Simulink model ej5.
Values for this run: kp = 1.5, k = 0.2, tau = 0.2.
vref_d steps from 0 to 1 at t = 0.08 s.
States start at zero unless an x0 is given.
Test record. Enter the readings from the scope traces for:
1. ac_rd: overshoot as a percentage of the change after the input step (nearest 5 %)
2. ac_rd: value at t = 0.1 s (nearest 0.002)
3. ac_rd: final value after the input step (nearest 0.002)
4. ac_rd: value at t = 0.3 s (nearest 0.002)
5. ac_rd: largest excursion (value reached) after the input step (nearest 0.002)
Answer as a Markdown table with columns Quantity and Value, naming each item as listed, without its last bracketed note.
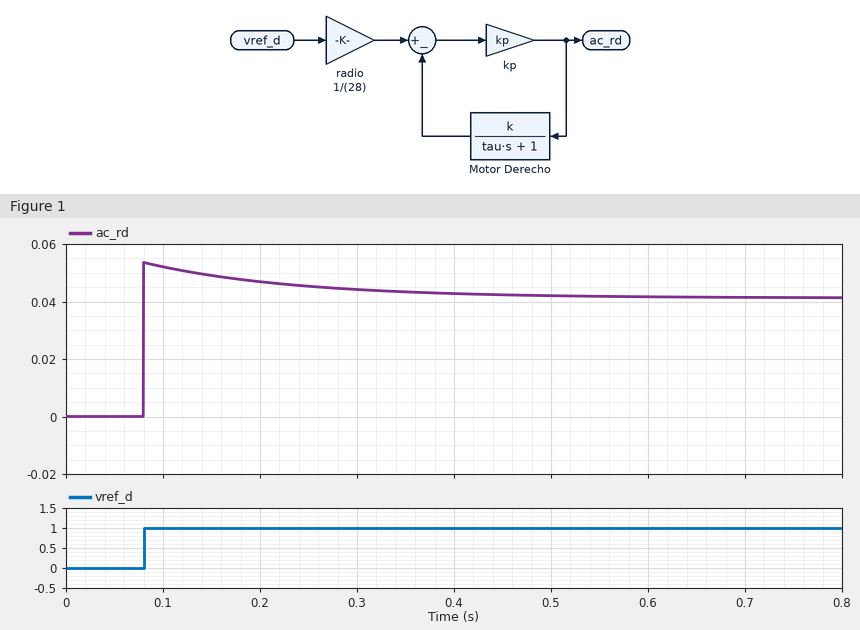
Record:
| Quantity | Value |
|---|---|
| ac_rd: overshoot as a percentage of the change after the input step | 30 % |
| ac_rd: value at t = 0.1 s | 0.052 |
| ac_rd: final value after the input step | 0.042 |
| ac_rd: value at t = 0.3 s | 0.044 |
| ac_rd: largest excursion (value reached) after the input step | 0.054 |
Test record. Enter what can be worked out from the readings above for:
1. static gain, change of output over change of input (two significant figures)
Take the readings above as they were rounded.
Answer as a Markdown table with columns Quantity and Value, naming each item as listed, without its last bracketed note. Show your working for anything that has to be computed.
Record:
| Quantity | Value |
|---|---|
| static gain, change of output over change of input | (0.042 - 0) / (1 - 0) = 0.042 |
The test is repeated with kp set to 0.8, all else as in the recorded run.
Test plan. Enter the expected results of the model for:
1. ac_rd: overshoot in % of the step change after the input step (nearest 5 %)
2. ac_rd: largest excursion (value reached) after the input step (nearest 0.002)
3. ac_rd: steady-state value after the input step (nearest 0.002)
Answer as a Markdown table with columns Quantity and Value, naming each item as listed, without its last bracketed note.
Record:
| Quantity | Value |
|---|---|
| ac_rd: overshoot in % of the step change after the input step | 15 % |
| ac_rd: largest excursion (value reached) after the input step | 0.028 |
| ac_rd: steady-state value after the input step | 0.024 |
